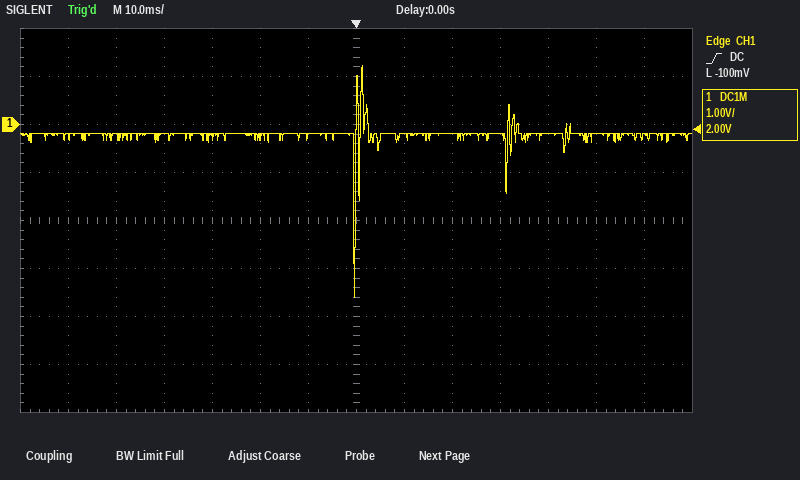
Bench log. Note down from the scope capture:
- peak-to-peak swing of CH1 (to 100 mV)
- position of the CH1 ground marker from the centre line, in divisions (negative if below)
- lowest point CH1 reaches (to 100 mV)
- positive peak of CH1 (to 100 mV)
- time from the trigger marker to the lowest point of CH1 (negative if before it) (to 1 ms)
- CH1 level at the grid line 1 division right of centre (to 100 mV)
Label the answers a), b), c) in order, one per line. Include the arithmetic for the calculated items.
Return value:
a) 1.2 V − (-3.6 V) = 4.8 V
b) +2.0 div
c) -3.6 V
d) 1.2 V
e) 0 ms
f) -200 mV
